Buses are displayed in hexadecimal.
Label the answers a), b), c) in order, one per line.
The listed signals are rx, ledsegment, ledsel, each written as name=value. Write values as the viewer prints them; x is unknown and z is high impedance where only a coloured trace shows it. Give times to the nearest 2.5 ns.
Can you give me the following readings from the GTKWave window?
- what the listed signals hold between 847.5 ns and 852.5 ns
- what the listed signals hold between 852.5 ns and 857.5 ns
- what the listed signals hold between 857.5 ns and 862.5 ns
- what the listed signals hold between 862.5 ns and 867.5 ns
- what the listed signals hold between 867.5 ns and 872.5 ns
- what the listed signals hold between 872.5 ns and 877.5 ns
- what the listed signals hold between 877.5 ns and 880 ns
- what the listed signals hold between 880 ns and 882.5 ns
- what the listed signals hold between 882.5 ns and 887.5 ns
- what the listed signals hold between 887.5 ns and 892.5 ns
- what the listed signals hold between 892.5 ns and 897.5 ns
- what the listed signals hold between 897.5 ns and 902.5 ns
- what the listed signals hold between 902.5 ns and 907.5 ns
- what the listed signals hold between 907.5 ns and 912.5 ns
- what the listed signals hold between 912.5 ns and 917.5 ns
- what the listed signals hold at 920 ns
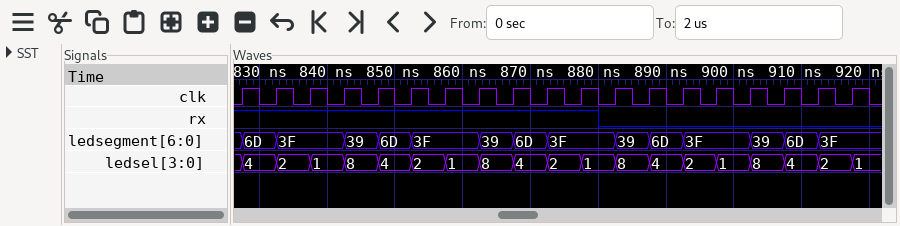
a) rx=1, ledsegment=6D, ledsel=4
b) rx=1, ledsegment=3F, ledsel=2
c) rx=1, ledsegment=3F, ledsel=1
d) rx=1, ledsegment=39, ledsel=8
e) rx=1, ledsegment=6D, ledsel=4
f) rx=1, ledsegment=3F, ledsel=2
g) rx=1, ledsegment=3F, ledsel=1
h) rx=0, ledsegment=3F, ledsel=1
i) rx=0, ledsegment=39, ledsel=8
j) rx=0, ledsegment=6D, ledsel=4
k) rx=0, ledsegment=3F, ledsel=2
l) rx=0, ledsegment=3F, ledsel=1
m) rx=0, ledsegment=39, ledsel=8
n) rx=0, ledsegment=6D, ledsel=4
o) rx=0, ledsegment=3F, ledsel=2
p) rx=0, ledsegment=3F, ledsel=1
